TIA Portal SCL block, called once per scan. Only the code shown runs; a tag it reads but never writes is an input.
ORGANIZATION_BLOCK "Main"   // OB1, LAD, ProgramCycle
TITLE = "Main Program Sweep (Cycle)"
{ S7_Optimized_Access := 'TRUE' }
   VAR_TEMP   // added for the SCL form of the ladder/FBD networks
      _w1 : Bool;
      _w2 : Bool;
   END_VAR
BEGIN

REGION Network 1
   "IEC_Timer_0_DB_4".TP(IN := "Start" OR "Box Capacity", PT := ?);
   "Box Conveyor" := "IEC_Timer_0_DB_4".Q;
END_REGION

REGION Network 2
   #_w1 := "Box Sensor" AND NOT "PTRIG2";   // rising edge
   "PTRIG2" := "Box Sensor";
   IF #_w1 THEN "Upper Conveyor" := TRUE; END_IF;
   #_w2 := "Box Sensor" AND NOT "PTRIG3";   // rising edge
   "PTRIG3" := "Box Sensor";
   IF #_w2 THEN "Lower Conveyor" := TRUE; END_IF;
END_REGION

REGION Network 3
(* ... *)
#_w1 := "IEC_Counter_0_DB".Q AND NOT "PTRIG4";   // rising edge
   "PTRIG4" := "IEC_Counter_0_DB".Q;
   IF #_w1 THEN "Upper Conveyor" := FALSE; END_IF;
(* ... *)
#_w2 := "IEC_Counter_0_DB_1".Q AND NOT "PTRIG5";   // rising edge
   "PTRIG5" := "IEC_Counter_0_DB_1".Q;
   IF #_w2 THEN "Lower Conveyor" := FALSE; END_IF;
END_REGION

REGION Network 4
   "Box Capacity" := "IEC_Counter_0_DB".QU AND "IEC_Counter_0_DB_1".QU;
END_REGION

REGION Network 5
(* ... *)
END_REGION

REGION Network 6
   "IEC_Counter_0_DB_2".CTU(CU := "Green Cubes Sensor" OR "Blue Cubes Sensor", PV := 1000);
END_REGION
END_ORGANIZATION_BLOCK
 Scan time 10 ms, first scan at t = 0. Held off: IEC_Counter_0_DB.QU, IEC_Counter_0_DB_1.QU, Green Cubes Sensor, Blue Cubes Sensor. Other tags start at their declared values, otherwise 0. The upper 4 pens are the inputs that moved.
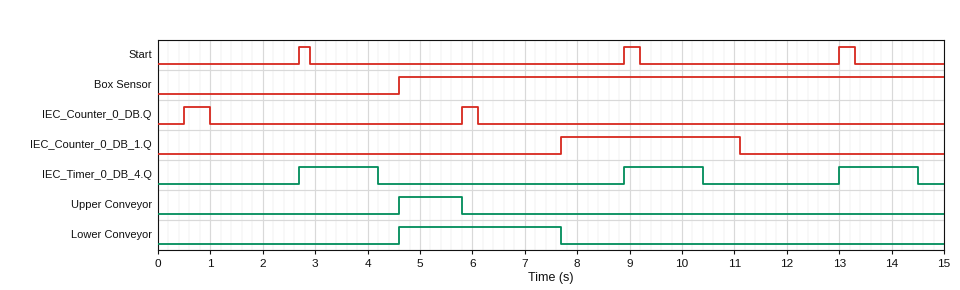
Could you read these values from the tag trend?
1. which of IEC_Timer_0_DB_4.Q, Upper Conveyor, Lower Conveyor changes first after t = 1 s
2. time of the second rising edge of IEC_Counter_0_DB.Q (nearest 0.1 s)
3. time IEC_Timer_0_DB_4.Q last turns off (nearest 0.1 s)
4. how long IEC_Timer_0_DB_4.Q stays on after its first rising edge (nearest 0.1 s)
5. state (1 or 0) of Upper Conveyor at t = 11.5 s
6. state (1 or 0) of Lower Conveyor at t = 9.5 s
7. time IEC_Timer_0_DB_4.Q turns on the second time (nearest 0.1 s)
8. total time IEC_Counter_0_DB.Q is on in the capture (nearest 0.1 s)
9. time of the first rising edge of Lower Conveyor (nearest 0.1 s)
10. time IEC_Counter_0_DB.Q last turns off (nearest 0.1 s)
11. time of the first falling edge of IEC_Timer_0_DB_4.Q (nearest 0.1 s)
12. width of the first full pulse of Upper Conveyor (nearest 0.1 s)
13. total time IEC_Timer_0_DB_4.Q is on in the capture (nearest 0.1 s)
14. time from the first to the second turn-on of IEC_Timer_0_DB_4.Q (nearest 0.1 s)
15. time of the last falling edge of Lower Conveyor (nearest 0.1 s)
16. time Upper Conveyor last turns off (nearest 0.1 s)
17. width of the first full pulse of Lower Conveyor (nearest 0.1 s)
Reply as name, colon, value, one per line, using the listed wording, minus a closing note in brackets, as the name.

which of IEC_Timer_0_DB_4.Q, Upper Conveyor, Lower Conveyor changes first after t = 1 s: IEC_Timer_0_DB_4.Q
time of the second rising edge of IEC_Counter_0_DB.Q: 5.8 s
time IEC_Timer_0_DB_4.Q last turns off: 14.5 s
how long IEC_Timer_0_DB_4.Q stays on after its first rising edge: 1.5 s
state (1 or 0) of Upper Conveyor at t = 11.5 s: 0
state (1 or 0) of Lower Conveyor at t = 9.5 s: 0
time IEC_Timer_0_DB_4.Q turns on the second time: 8.9 s
total time IEC_Counter_0_DB.Q is on in the capture: 0.8 s
time of the first rising edge of Lower Conveyor: 4.6 s
time IEC_Counter_0_DB.Q last turns off: 6.1 s
time of the first falling edge of IEC_Timer_0_DB_4.Q: 4.2 s
width of the first full pulse of Upper Conveyor: 1.2 s
total time IEC_Timer_0_DB_4.Q is on in the capture: 4.5 s
time from the first to the second turn-on of IEC_Timer_0_DB_4.Q: 6.2 s
time of the last falling edge of Lower Conveyor: 7.7 s
time Upper Conveyor last turns off: 5.8 s
width of the first full pulse of Lower Conveyor: 3.1 s
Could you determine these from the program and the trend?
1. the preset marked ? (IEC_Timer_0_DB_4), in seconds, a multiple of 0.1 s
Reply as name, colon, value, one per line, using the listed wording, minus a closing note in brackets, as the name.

the preset marked ? (IEC_Timer_0_DB_4), in seconds, a multiple of 0.1 s: 1.5 s
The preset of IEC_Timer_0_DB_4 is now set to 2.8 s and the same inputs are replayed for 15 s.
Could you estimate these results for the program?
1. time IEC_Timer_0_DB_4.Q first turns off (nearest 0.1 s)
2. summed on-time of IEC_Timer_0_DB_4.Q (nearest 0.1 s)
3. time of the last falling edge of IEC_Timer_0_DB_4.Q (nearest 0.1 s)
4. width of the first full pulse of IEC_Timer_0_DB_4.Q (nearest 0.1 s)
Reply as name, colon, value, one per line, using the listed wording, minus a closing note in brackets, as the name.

time IEC_Timer_0_DB_4.Q first turns off: 5.5 s
summed on-time of IEC_Timer_0_DB_4.Q: 7.6 s
time of the last falling edge of IEC_Timer_0_DB_4.Q: 11.7 s
width of the first full pulse of IEC_Timer_0_DB_4.Q: 2.8 s
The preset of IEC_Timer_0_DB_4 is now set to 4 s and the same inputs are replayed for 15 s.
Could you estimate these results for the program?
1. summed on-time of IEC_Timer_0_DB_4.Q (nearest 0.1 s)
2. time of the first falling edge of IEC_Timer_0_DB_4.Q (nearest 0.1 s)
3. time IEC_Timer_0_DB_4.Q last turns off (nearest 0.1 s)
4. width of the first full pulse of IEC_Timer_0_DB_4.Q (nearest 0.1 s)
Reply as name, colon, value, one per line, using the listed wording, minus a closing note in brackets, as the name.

summed on-time of IEC_Timer_0_DB_4.Q: 10.0 s
time of the first falling edge of IEC_Timer_0_DB_4.Q: 6.7 s
time IEC_Timer_0_DB_4.Q last turns off: 12.9 s
width of the first full pulse of IEC_Timer_0_DB_4.Q: 4.0 s
